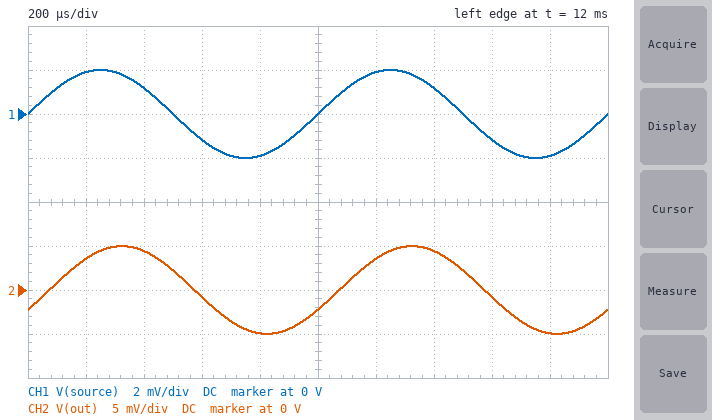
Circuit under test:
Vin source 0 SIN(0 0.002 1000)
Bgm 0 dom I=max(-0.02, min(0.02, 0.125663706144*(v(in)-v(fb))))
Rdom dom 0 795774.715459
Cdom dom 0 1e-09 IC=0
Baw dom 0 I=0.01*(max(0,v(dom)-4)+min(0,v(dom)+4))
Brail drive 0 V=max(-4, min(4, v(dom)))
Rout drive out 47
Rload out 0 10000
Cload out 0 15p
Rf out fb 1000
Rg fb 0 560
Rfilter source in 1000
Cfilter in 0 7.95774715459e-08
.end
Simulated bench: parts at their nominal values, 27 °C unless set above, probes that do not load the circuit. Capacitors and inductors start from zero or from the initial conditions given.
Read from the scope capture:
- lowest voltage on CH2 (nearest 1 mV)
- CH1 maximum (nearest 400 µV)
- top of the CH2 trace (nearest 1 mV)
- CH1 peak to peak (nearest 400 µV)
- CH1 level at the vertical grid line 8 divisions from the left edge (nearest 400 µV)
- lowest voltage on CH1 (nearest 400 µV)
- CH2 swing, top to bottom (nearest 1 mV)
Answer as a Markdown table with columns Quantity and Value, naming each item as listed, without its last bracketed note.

| Quantity | Value |
|---|---|
| lowest voltage on CH2 | -5 mV |
| CH1 maximum | 2.0 mV |
| top of the CH2 trace | 5 mV |
| CH1 peak to peak | 4.0 mV |
| CH1 level at the vertical grid line 8 divisions from the left edge | -1.2 mV |
| lowest voltage on CH1 | -2.0 mV |
| CH2 swing, top to bottom | 10 mV |
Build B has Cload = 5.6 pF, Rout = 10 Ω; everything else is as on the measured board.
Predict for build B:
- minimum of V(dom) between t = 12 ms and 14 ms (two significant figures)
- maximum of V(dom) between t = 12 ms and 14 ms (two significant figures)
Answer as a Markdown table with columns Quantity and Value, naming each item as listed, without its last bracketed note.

| Quantity | Value |
|---|---|
| minimum of V(dom) between t = 12 ms and 14 ms | -5.0 mV |
| maximum of V(dom) between t = 12 ms and 14 ms | 5.0 mV |
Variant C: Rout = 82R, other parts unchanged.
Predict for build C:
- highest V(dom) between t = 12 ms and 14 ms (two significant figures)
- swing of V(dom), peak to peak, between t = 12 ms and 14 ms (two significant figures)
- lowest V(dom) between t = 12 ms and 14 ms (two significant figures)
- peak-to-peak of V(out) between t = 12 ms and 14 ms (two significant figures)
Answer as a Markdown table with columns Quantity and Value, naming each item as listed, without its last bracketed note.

| Quantity | Value |
|---|---|
| highest V(dom) between t = 12 ms and 14 ms | 5.3 mV |
| swing of V(dom), peak to peak, between t = 12 ms and 14 ms | 11 mV |
| lowest V(dom) between t = 12 ms and 14 ms | -5.3 mV |
| peak-to-peak of V(out) between t = 12 ms and 14 ms | 10 mV |
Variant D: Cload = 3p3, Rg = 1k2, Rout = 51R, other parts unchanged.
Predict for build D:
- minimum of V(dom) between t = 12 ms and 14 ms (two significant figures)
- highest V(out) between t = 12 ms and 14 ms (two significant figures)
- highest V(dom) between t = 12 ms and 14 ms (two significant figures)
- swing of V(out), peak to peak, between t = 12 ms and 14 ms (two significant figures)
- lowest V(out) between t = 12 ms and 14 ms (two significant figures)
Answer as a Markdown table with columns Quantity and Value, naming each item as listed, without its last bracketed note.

| Quantity | Value |
|---|---|
| minimum of V(dom) between t = 12 ms and 14 ms | -3.4 mV |
| highest V(out) between t = 12 ms and 14 ms | 3.3 mV |
| highest V(dom) between t = 12 ms and 14 ms | 3.4 mV |
| swing of V(out), peak to peak, between t = 12 ms and 14 ms | 6.6 mV |
| lowest V(out) between t = 12 ms and 14 ms | -3.3 mV |
